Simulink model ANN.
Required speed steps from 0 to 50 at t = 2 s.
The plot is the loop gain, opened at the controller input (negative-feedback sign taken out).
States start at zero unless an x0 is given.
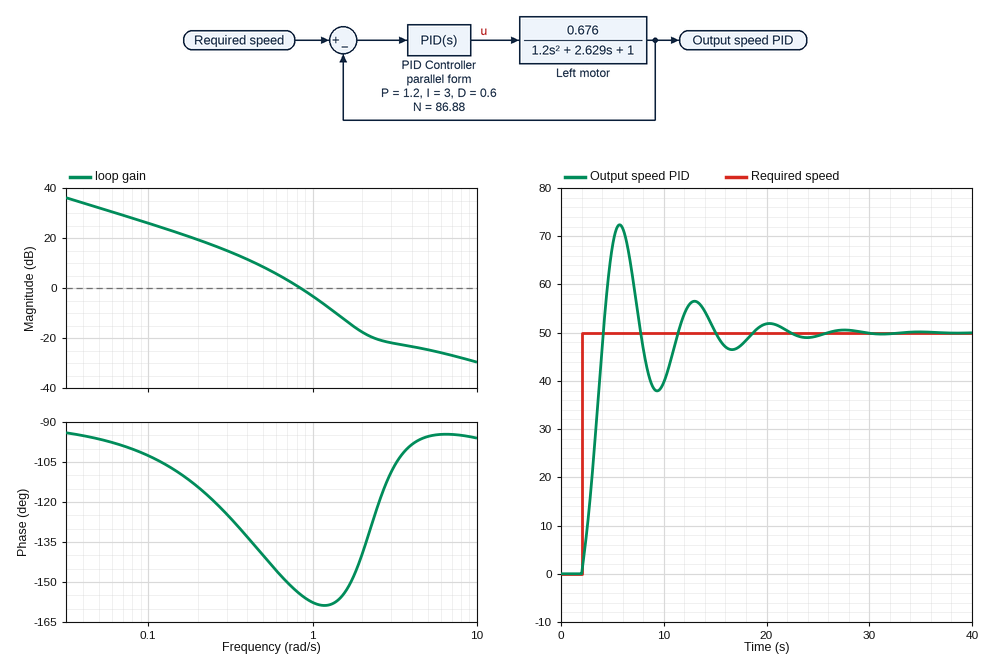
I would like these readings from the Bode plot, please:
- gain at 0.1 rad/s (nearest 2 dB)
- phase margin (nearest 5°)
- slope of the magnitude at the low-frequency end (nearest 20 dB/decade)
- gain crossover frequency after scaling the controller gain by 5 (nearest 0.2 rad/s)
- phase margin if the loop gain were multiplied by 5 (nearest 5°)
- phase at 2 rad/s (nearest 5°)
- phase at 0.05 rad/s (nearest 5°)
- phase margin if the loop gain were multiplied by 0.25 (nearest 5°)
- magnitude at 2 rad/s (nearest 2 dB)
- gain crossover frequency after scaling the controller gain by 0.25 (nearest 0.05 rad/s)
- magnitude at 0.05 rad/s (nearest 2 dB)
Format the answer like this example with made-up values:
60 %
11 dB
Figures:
26 dB
25°
-20 dB/decade
1.6 rad/s
30°
-140°
-95°
50°
-18 dB
0.40 rad/s
32 dB
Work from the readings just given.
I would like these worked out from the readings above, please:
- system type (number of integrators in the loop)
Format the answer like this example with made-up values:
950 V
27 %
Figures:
1
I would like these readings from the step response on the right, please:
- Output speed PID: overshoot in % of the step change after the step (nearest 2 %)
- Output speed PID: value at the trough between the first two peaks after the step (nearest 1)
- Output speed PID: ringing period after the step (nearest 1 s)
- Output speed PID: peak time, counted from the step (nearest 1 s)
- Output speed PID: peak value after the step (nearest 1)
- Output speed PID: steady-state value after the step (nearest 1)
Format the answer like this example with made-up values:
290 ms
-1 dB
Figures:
44 %
38
7 s
4 s
72
50
